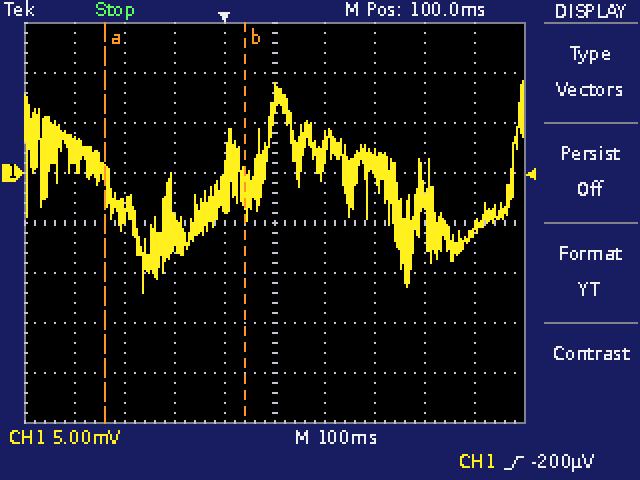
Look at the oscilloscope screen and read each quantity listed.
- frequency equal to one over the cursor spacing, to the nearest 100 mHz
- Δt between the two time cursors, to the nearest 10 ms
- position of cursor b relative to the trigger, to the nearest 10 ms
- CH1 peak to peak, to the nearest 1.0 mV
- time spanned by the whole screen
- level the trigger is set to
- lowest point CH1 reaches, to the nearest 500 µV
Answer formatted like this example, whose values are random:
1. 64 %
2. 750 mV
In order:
1. 3.6 Hz
2. 280 ms
3. +40 ms
4. 21.0 mV
5. 1 s
6. -200 µV
7. -12.0 mV
